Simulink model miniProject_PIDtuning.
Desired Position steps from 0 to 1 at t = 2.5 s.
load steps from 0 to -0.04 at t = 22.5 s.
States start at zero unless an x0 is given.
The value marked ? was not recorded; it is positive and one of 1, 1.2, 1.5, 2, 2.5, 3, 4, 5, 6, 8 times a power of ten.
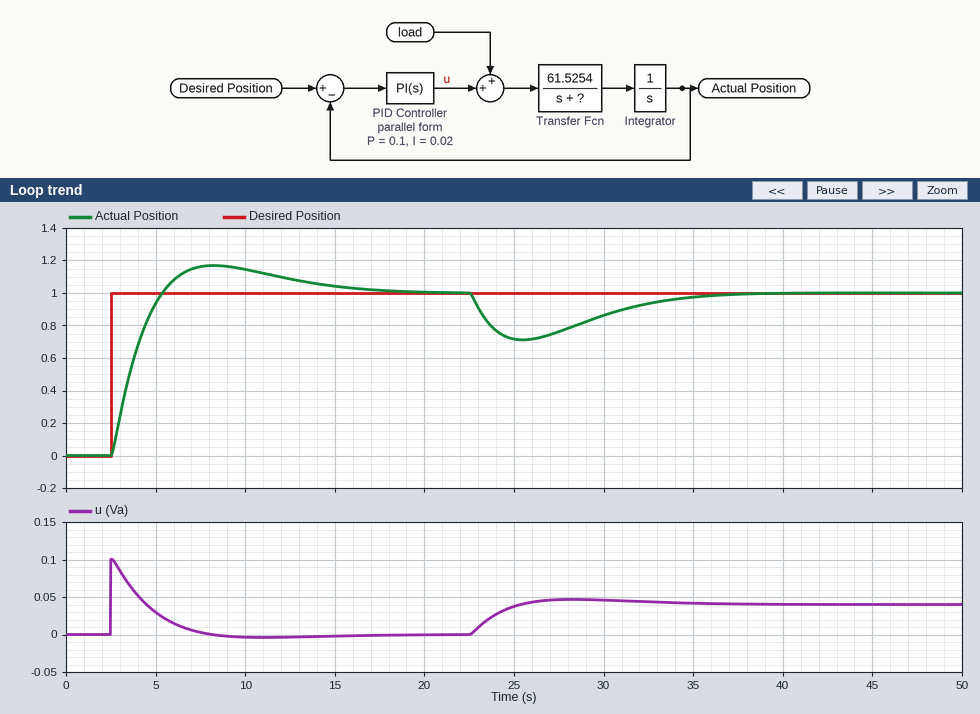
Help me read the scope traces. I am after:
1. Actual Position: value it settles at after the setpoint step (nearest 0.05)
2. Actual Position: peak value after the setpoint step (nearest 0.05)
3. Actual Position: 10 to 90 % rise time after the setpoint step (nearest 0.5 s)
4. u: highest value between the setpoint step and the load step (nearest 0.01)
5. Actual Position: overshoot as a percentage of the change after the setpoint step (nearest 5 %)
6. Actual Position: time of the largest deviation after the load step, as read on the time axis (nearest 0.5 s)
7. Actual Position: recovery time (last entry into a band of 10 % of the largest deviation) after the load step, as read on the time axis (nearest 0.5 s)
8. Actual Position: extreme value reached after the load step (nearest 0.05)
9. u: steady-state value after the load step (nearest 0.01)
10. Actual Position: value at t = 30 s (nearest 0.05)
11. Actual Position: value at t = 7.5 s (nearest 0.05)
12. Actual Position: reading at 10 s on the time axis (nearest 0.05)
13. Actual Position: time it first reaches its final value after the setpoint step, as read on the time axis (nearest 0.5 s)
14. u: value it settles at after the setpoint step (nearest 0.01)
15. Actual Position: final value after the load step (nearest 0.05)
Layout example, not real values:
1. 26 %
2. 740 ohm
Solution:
1. 1.00
2. 1.15
3. 2.0 s
4. 0.10
5. 15 %
6. 25.5 s
7. 34.5 s
8. 0.70
9. 0.04
10. 0.85
11. 1.15
12. 1.15
13. 5.5 s
14. 0.00
15. 1.00
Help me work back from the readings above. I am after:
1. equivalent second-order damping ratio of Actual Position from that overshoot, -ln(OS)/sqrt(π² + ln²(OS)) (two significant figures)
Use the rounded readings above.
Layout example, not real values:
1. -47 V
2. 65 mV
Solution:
1. 0.52
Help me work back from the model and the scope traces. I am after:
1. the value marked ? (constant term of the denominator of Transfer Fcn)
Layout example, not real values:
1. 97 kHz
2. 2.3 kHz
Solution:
1. 10
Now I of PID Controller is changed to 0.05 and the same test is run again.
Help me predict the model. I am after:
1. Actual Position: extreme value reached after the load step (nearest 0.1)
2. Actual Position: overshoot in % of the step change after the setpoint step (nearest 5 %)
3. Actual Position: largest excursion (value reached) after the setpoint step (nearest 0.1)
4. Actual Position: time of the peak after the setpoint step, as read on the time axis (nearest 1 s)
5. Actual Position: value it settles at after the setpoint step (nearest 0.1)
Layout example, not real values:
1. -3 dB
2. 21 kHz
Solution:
1. 0.8
2. 30 %
3. 1.3
4. 7 s
5. 1.0
